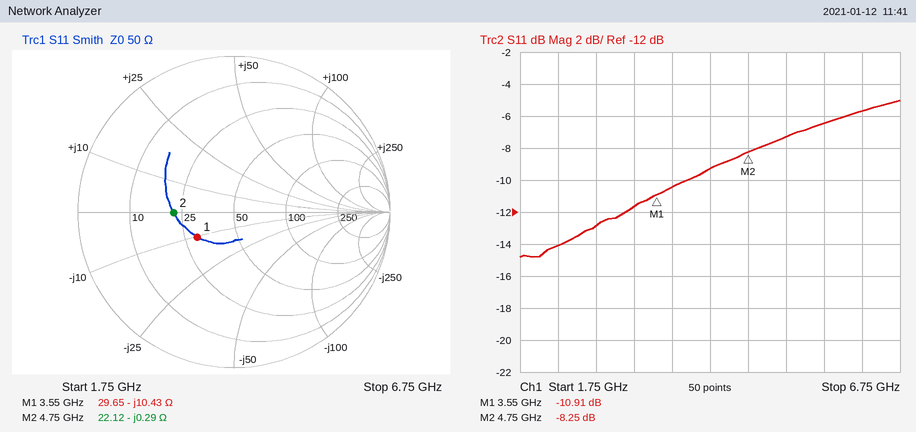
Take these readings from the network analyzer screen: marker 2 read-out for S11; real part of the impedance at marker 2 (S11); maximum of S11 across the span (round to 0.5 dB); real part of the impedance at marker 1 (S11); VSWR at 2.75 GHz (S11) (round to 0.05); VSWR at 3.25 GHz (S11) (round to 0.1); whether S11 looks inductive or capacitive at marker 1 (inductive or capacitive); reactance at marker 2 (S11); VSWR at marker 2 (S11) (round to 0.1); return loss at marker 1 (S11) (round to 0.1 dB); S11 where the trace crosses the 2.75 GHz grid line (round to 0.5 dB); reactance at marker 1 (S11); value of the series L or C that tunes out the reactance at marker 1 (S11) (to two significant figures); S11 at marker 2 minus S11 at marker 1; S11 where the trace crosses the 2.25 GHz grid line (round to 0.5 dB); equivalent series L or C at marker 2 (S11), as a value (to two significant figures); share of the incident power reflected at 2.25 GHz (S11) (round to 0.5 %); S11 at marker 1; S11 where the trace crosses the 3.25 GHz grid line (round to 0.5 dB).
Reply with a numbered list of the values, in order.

1. -8.25 dB
2. 22.12 Ω
3. -5.0 dB
4. 29.65 Ω
5. 1.60
6. 1.7
7. capacitive
8. -0.29 Ω
9. 2.3
10. 10.9 dB
11. -13.0 dB
12. -10.43 Ω
13. 470 pH
14. 2.66 dB
15. -14.0 dB
16. 120 pF
17. 4.0 %
18. -10.91 dB
19. -11.5 dB
